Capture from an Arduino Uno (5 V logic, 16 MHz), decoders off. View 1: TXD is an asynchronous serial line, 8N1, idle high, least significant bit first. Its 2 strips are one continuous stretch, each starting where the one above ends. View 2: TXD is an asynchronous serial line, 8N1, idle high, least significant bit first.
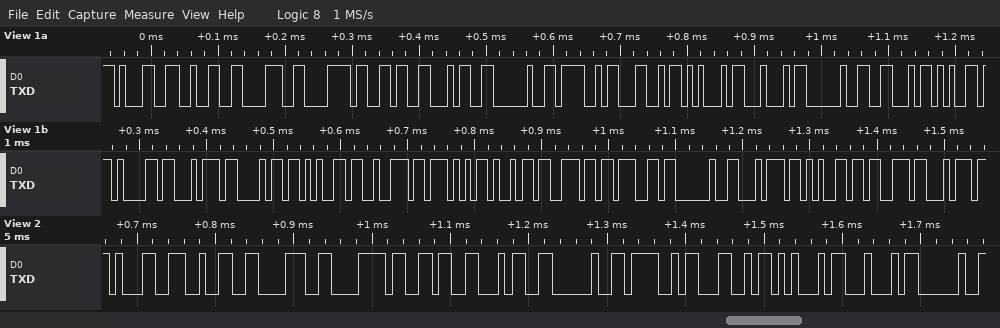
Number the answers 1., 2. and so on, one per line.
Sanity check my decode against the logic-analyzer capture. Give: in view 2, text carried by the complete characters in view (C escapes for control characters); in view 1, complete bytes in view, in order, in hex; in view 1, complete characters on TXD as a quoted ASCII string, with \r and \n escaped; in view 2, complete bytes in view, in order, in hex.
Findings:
1. "128x64 OLED "
2. 31 32 38 78 36 34 20 4F 4C 45 44 20 46 65 61 74 68 65 72 57 69 6E 67 20 74 65 73 74
3. "128x64 OLED FeatherWing test"
4. 31 32 38 78 36 34 20 4F 4C 45 44 20
